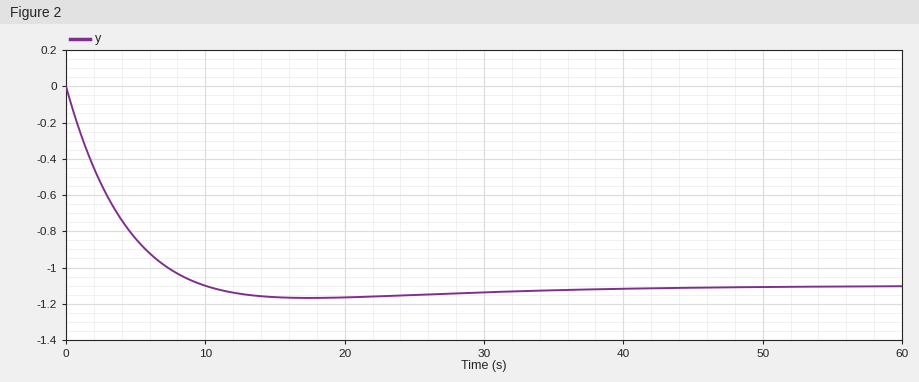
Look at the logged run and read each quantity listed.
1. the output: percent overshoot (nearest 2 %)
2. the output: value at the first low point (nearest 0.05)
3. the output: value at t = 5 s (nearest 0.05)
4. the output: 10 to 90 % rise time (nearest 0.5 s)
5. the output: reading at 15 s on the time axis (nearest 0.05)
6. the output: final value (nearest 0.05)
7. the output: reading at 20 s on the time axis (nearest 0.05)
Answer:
6 %
-1.15
-0.85
6.5 s
-1.15
-1.10
-1.15
